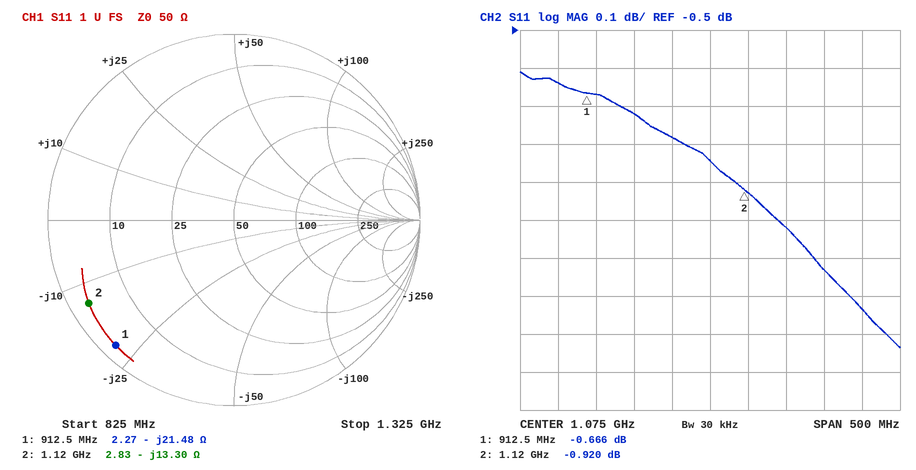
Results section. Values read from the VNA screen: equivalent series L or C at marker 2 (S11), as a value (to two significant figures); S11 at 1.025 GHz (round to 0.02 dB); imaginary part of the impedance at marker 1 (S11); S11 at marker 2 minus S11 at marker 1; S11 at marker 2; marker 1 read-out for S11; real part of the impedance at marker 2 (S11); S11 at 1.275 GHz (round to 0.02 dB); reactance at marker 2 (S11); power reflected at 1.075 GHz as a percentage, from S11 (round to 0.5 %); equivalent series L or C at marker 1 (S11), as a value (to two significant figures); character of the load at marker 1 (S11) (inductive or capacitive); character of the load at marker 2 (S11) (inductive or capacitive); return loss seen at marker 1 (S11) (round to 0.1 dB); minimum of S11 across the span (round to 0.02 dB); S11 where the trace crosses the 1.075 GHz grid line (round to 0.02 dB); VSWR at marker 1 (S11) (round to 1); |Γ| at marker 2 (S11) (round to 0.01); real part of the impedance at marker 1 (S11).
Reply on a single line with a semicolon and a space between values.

11 pF; -0.78 dB; -21.48 Ω; -0.254 dB; -0.920 dB; -0.666 dB; 2.83 Ω; -1.24 dB; -13.30 Ω; 82.5 %; 8.1 pF; capacitive; capacitive; 0.7 dB; -1.34 dB; -0.84 dB; 26; 0.90; 2.27 Ω
